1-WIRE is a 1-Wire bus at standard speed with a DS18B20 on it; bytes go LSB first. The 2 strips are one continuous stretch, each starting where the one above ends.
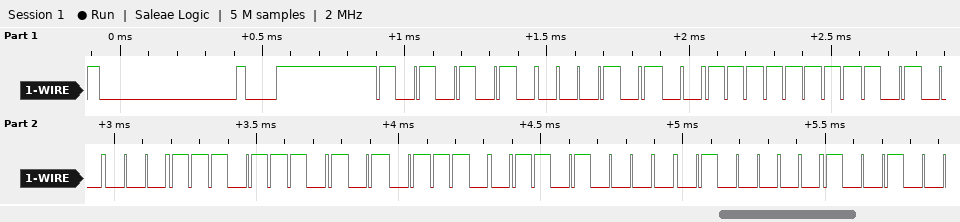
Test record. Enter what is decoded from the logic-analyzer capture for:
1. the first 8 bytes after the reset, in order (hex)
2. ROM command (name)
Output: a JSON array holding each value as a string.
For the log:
["55 28 FF 05 77 75 16 04", "Match ROM"]
